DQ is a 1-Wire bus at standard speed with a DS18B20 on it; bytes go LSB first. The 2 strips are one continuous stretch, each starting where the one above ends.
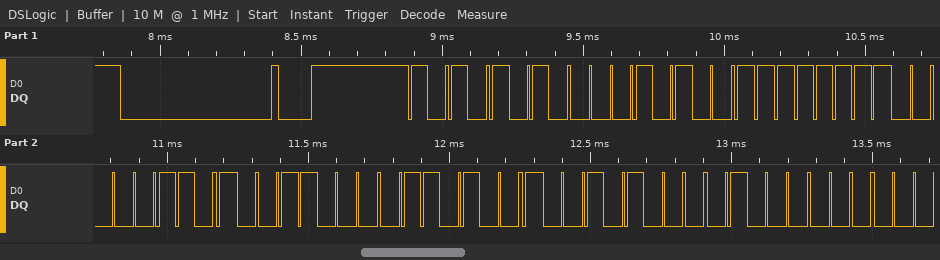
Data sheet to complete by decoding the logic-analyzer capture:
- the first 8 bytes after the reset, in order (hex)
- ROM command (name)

55 28 FF 60 19 96 14 02
Match ROM
